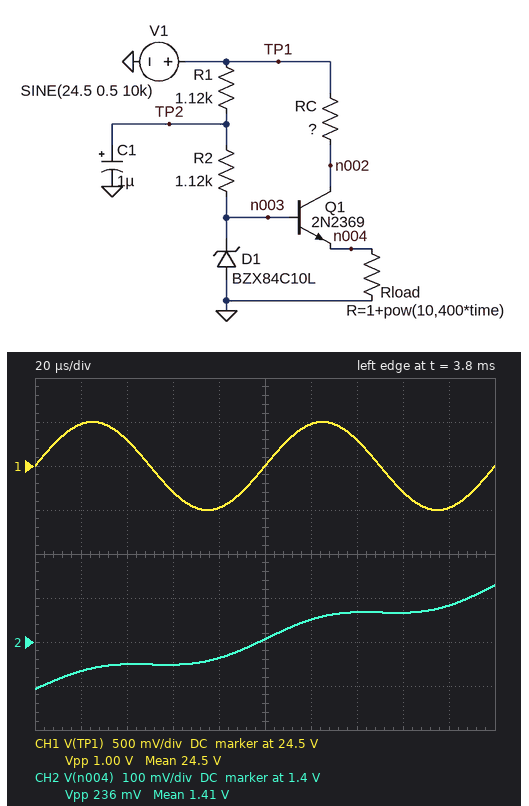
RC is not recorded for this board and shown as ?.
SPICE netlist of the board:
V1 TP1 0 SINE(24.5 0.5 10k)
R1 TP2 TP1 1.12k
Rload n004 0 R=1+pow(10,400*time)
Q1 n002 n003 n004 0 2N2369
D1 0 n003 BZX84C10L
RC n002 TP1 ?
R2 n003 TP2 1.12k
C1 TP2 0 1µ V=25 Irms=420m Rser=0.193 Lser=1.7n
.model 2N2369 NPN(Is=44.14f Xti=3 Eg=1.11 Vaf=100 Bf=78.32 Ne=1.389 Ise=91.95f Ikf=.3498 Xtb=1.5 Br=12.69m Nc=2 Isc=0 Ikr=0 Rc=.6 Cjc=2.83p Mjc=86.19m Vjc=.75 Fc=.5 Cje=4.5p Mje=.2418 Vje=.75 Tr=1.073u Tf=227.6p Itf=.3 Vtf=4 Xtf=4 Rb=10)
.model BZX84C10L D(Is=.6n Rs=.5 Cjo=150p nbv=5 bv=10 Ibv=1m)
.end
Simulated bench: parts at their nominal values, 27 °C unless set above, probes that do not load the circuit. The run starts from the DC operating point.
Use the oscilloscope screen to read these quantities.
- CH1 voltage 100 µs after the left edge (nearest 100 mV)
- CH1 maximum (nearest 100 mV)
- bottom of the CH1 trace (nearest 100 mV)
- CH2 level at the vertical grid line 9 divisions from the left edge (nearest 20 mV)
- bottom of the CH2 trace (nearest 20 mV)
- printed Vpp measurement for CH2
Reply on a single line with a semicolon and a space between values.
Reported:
24.5 V; 25.0 V; 24.0 V; 1.48 V; 1.30 V; 236 mV
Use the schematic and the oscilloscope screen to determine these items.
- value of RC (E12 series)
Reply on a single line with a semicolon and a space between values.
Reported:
820 Ω
